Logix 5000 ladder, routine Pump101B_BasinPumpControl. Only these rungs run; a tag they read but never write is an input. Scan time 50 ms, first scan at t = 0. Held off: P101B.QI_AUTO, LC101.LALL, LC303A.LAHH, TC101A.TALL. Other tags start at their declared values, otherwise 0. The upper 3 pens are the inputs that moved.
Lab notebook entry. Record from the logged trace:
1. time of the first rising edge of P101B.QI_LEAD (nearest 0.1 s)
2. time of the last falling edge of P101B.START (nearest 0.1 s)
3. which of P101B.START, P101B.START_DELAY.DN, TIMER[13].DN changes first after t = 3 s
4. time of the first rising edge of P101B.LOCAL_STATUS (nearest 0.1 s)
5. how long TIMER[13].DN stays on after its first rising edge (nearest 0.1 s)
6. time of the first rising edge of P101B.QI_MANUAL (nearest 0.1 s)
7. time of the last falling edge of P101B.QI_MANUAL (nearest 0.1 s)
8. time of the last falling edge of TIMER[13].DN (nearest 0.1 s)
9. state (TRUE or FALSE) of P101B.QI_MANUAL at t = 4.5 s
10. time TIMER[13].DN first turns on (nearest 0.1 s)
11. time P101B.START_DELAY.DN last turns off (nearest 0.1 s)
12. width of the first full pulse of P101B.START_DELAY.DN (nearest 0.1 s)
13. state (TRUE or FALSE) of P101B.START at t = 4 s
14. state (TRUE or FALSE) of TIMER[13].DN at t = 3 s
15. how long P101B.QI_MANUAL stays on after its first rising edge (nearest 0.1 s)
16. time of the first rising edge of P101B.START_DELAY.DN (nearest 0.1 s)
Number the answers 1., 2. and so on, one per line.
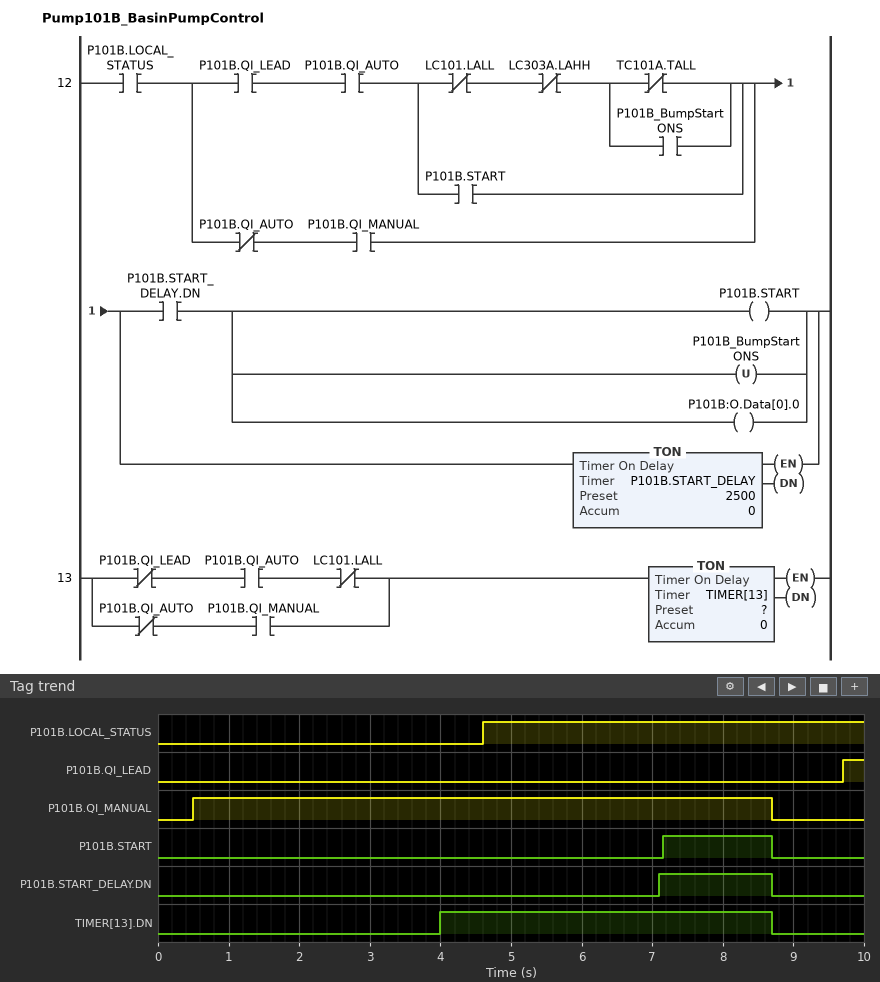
1. 9.7 s
2. 8.7 s
3. TIMER[13].DN
4. 4.6 s
5. 4.7 s
6. 0.5 s
7. 8.7 s
8. 8.7 s
9. TRUE
10. 4.0 s
11. 8.7 s
12. 1.6 s
13. FALSE
14. FALSE
15. 8.2 s
16. 7.1 s
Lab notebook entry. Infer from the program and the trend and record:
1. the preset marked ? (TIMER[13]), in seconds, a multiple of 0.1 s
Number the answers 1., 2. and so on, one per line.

1. 3.5 s
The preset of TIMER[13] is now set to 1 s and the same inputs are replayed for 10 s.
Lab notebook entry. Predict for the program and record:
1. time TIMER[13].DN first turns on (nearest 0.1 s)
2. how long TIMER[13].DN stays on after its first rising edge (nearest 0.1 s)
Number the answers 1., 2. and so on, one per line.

1. 1.5 s
2. 7.2 s
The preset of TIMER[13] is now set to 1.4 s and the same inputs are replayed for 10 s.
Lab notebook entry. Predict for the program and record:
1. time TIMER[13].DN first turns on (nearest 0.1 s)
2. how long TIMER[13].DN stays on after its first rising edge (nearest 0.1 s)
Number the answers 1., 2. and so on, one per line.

1. 1.9 s
2. 6.8 s
